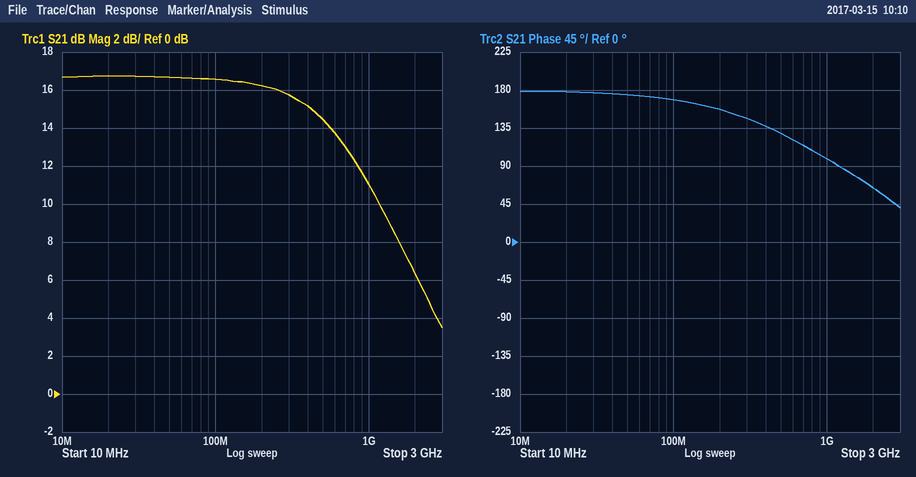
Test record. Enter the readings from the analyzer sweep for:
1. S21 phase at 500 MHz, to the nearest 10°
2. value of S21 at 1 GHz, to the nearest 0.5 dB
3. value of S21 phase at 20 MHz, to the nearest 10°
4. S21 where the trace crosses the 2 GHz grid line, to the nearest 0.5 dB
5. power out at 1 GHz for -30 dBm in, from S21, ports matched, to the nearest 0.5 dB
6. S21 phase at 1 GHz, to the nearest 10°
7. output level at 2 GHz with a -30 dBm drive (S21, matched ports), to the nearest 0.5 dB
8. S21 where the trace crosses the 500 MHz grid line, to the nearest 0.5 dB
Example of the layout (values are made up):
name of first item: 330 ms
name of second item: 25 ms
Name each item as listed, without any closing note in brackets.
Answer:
S21 phase at 500 MHz, to the nearest 10°: 130°
value of S21 at 1 GHz, to the nearest 0.5 dB: 11.0 dB
value of S21 phase at 20 MHz, to the nearest 10°: 180°
S21 where the trace crosses the 2 GHz grid line, to the nearest 0.5 dB: 6.5 dB
power out at 1 GHz for -30 dBm in, from S21, ports matched, to the nearest 0.5 dB: -19.0 dBm
S21 phase at 1 GHz, to the nearest 10°: 100°
output level at 2 GHz with a -30 dBm drive (S21, matched ports), to the nearest 0.5 dB: -23.5 dBm
S21 where the trace crosses the 500 MHz grid line, to the nearest 0.5 dB: 14.5 dB
